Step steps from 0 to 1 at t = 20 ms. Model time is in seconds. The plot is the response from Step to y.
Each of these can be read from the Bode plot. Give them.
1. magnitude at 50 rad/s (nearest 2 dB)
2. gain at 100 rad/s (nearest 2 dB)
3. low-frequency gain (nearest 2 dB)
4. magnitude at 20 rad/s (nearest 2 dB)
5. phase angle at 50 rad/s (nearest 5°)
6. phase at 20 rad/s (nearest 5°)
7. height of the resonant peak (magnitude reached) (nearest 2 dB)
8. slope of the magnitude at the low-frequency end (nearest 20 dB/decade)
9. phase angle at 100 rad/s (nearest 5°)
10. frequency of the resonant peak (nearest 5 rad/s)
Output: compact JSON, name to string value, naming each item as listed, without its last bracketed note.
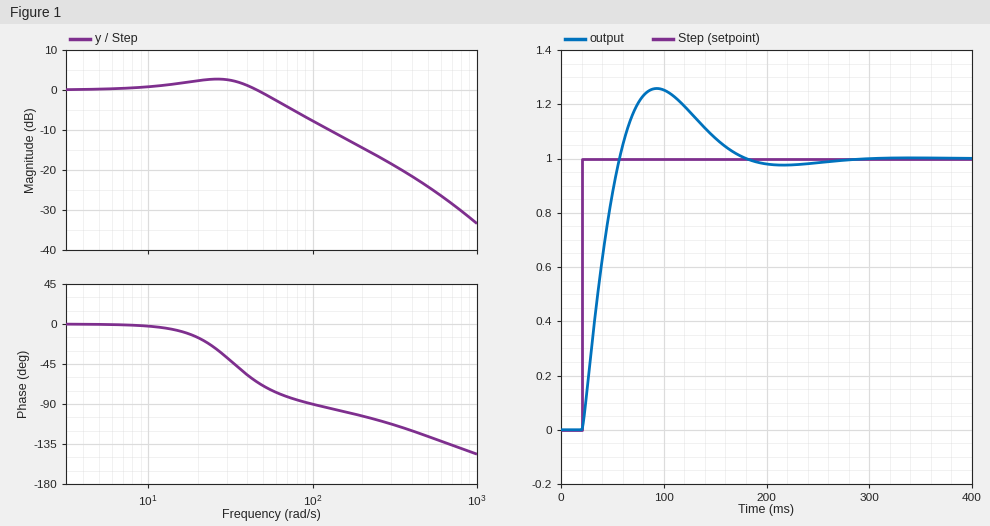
{"magnitude at 50 rad/s": "0 dB", "gain at 100 rad/s": "-8 dB", "low-frequency gain": "0 dB", "magnitude at 20 rad/s": "2 dB", "phase angle at 50 rad/s": "-70°", "phase at 20 rad/s": "-15°", "height of the resonant peak (magnitude reached)": "2 dB", "slope of the magnitude at the low-frequency end": "0 dB/decade", "phase angle at 100 rad/s": "-90°", "frequency of the resonant peak": "25 rad/s"}
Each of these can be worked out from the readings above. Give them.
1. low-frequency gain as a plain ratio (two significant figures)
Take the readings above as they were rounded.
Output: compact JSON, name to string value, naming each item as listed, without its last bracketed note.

{"low-frequency gain as a plain ratio": "1.0"}
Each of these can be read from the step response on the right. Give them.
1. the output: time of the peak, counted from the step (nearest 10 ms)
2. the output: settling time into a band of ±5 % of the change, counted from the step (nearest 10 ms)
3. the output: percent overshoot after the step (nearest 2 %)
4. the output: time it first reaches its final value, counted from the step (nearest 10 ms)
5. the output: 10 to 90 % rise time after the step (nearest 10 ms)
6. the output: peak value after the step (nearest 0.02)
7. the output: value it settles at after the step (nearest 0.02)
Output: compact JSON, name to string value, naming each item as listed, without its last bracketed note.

{"the output: time of the peak, counted from the step": "70 ms", "the output: settling time into a band of ±5 % of the change, counted from the step": "140 ms", "the output: percent overshoot after the step": "26 %", "the output: time it first reaches its final value, counted from the step": "40 ms", "the output: 10 to 90 % rise time after the step": "30 ms", "the output: peak value after the step": "1.26", "the output: value it settles at after the step": "1.00"}
